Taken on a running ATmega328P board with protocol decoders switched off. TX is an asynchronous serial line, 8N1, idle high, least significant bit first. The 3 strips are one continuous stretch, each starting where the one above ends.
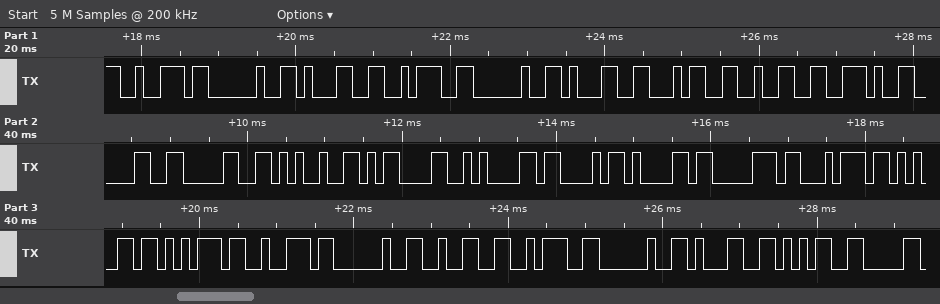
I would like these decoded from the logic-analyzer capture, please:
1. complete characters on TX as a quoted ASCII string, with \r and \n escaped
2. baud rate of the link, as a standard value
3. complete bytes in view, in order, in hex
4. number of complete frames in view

"r 1: 142.00%\r\nCapteur 2: 15"
9600 baud
72 20 31 3A 20 31 34 32 2E 30 30 25 0D 0A 43 61 70 74 65 75 72 20 32 3A 20 31 35
27
